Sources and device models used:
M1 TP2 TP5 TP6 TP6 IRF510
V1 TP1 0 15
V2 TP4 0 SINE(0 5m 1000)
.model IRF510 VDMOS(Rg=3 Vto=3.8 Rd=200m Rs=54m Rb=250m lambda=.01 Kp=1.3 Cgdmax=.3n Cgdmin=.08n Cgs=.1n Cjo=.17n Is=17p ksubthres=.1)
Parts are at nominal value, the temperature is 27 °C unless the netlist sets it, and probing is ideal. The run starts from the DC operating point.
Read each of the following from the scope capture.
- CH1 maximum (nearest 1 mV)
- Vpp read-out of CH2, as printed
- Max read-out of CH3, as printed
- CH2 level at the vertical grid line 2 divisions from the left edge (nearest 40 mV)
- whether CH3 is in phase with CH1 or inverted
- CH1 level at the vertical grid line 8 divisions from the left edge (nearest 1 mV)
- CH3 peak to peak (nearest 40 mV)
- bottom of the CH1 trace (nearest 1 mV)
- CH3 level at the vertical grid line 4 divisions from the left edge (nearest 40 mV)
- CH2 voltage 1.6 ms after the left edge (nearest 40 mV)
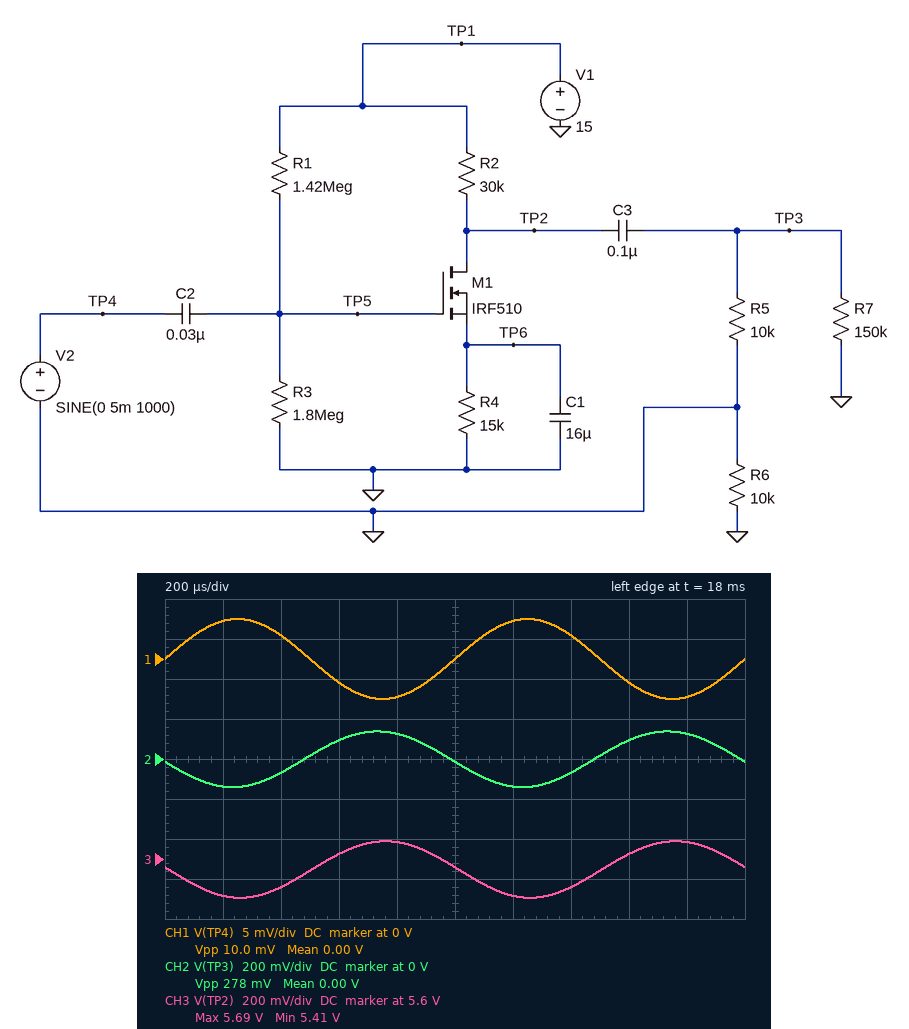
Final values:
5 mV
278 mV
5.69 V
-80 mV
inverted
-3 mV
280 mV
-5 mV
5.68 V
80 mV
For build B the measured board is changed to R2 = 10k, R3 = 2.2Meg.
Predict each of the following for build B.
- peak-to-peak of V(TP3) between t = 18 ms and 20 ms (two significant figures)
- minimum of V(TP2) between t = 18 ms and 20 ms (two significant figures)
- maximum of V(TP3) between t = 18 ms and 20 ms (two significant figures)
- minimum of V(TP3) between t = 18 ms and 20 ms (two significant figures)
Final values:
270 mV
11 V
130 mV
-140 mV
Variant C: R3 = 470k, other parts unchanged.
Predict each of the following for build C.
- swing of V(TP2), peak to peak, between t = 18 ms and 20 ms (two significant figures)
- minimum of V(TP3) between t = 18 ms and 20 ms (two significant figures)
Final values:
22 mV
-11 mV
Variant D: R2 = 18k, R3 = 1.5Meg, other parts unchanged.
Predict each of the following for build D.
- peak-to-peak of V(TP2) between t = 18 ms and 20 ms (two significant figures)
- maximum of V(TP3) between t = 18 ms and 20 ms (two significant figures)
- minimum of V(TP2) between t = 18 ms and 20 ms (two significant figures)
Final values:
270 mV
130 mV
10 V
